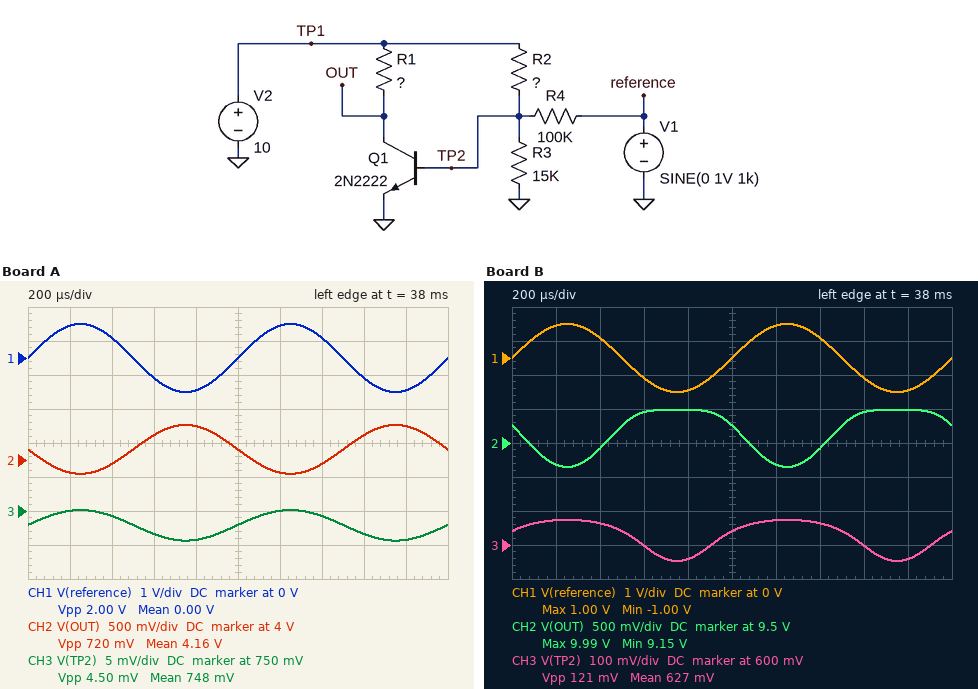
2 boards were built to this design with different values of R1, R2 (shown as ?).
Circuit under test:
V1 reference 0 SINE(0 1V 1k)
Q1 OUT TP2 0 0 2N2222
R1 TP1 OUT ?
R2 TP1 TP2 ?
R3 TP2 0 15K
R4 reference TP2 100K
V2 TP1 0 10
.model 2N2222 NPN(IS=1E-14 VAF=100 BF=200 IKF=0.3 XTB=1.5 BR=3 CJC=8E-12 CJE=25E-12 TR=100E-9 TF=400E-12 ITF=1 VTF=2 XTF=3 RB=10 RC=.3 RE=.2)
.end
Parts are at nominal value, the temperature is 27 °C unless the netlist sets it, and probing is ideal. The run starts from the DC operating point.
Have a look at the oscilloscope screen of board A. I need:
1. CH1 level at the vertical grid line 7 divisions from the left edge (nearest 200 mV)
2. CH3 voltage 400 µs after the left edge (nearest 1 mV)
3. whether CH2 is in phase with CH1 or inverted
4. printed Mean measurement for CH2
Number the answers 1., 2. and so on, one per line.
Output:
1. 600 mV
2. 749 mV
3. inverted
4. 4.16 V
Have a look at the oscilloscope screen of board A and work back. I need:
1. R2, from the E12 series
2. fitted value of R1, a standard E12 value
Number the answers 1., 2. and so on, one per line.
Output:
1. 47 kΩ
2. 220 Ω
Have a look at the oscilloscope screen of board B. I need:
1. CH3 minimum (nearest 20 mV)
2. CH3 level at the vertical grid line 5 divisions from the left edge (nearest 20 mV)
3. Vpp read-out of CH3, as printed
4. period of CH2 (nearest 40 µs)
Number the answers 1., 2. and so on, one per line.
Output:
1. 560 mV
2. 640 mV
3. 121 mV
4. 1.00 ms
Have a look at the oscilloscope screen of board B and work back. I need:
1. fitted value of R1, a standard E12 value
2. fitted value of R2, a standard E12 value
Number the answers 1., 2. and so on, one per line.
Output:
1. 390 Ω
2. 180 kΩ
